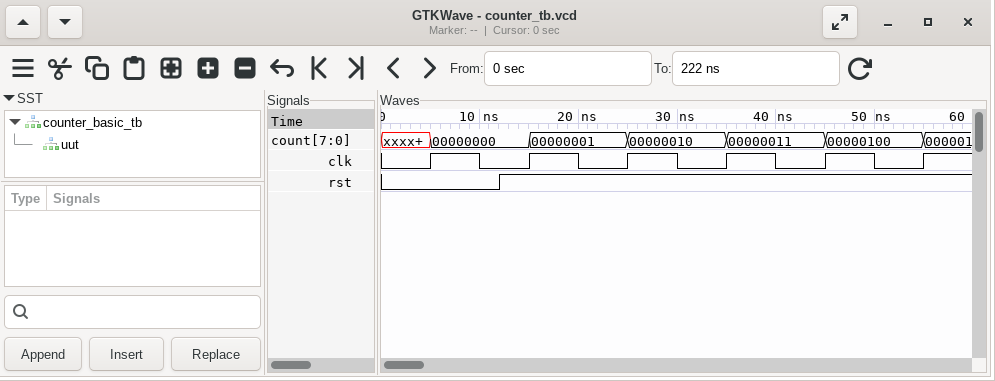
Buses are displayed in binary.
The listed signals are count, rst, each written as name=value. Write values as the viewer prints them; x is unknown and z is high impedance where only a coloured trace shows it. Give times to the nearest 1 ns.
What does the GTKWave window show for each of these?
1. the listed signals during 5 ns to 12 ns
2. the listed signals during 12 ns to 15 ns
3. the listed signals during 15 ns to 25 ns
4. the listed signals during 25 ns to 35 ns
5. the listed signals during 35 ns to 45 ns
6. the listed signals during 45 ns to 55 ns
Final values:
count=00000000, rst=0
count=00000000, rst=1
count=00000001, rst=1
count=00000010, rst=1
count=00000011, rst=1
count=00000100, rst=1
